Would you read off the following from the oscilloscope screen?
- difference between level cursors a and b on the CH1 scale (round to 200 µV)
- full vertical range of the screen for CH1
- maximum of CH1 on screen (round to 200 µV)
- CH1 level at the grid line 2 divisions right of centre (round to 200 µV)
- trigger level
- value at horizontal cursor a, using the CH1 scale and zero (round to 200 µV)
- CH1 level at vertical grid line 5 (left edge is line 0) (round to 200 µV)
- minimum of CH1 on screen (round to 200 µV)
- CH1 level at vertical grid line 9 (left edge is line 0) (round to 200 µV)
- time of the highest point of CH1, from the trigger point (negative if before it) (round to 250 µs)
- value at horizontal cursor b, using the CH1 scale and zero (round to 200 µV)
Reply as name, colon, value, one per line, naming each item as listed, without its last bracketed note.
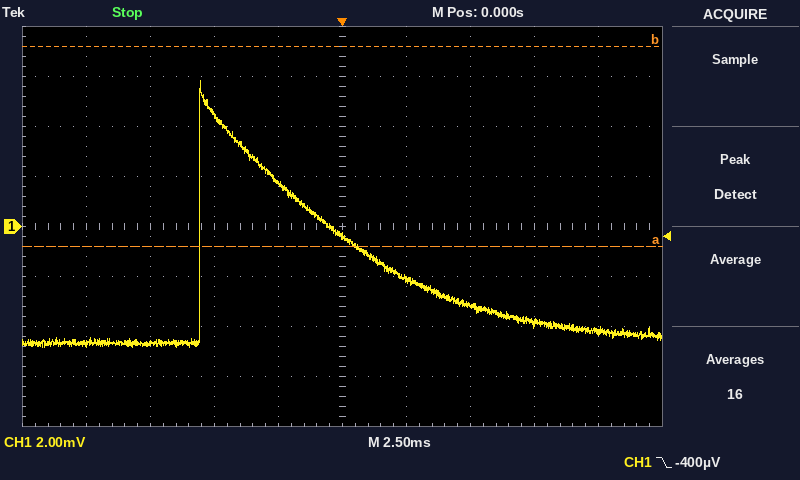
difference between level cursors a and b on the CH1 scale: 8.0 mV
full vertical range of the screen for CH1: 16 mV
maximum of CH1 on screen: 5.8 mV
CH1 level at the grid line 2 divisions right of centre: -3.2 mV
trigger level: -400 µV
value at horizontal cursor a, using the CH1 scale and zero: -800 µV
CH1 level at vertical grid line 5 (left edge is line 0): -400 µV
minimum of CH1 on screen: -4.8 mV
CH1 level at vertical grid line 9 (left edge is line 0): -4.2 mV
time of the highest point of CH1, from the trigger point (negative if before it): -5.50 ms
value at horizontal cursor b, using the CH1 scale and zero: 7.2 mV
